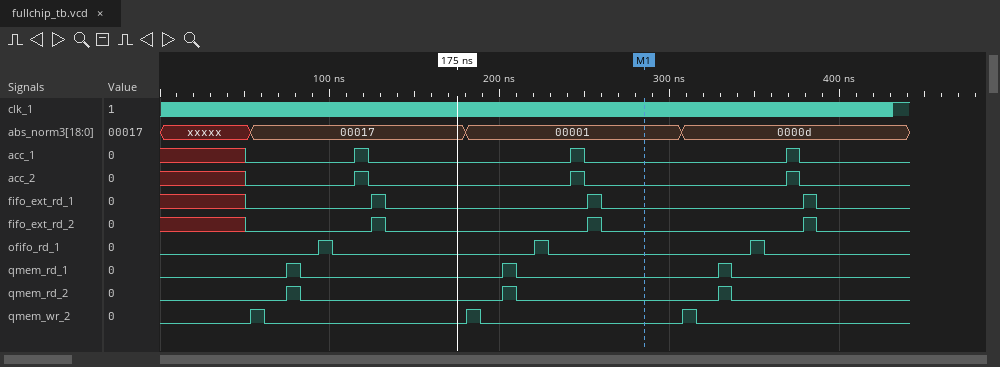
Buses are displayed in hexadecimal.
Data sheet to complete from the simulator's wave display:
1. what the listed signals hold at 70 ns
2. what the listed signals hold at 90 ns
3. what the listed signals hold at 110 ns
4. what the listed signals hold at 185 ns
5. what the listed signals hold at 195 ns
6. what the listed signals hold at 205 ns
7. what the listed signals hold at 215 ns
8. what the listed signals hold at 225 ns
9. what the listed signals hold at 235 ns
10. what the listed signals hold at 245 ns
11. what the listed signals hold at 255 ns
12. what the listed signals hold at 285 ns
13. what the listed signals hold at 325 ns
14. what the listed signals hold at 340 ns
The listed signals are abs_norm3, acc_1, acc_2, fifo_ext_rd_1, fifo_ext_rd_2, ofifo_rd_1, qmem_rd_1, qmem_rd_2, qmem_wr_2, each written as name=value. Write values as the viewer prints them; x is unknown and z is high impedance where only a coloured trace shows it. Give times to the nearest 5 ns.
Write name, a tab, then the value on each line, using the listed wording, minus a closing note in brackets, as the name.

what the listed signals hold at 70 ns	abs_norm3=00017, acc_1=0, acc_2=0, fifo_ext_rd_1=0, fifo_ext_rd_2=0, ofifo_rd_1=0, qmem_rd_1=0, qmem_rd_2=0, qmem_wr_2=0
what the listed signals hold at 90 ns	abs_norm3=00017, acc_1=0, acc_2=0, fifo_ext_rd_1=0, fifo_ext_rd_2=0, ofifo_rd_1=0, qmem_rd_1=0, qmem_rd_2=0, qmem_wr_2=0
what the listed signals hold at 110 ns	abs_norm3=00017, acc_1=0, acc_2=0, fifo_ext_rd_1=0, fifo_ext_rd_2=0, ofifo_rd_1=0, qmem_rd_1=0, qmem_rd_2=0, qmem_wr_2=0
what the listed signals hold at 185 ns	abs_norm3=00001, acc_1=0, acc_2=0, fifo_ext_rd_1=0, fifo_ext_rd_2=0, ofifo_rd_1=0, qmem_rd_1=0, qmem_rd_2=0, qmem_wr_2=1
what the listed signals hold at 195 ns	abs_norm3=00001, acc_1=0, acc_2=0, fifo_ext_rd_1=0, fifo_ext_rd_2=0, ofifo_rd_1=0, qmem_rd_1=0, qmem_rd_2=0, qmem_wr_2=0
what the listed signals hold at 205 ns	abs_norm3=00001, acc_1=0, acc_2=0, fifo_ext_rd_1=0, fifo_ext_rd_2=0, ofifo_rd_1=0, qmem_rd_1=1, qmem_rd_2=1, qmem_wr_2=0
what the listed signals hold at 215 ns	abs_norm3=00001, acc_1=0, acc_2=0, fifo_ext_rd_1=0, fifo_ext_rd_2=0, ofifo_rd_1=0, qmem_rd_1=0, qmem_rd_2=0, qmem_wr_2=0
what the listed signals hold at 225 ns	abs_norm3=00001, acc_1=0, acc_2=0, fifo_ext_rd_1=0, fifo_ext_rd_2=0, ofifo_rd_1=1, qmem_rd_1=0, qmem_rd_2=0, qmem_wr_2=0
what the listed signals hold at 235 ns	abs_norm3=00001, acc_1=0, acc_2=0, fifo_ext_rd_1=0, fifo_ext_rd_2=0, ofifo_rd_1=0, qmem_rd_1=0, qmem_rd_2=0, qmem_wr_2=0
what the listed signals hold at 245 ns	abs_norm3=00001, acc_1=1, acc_2=1, fifo_ext_rd_1=0, fifo_ext_rd_2=0, ofifo_rd_1=0, qmem_rd_1=0, qmem_rd_2=0, qmem_wr_2=0
what the listed signals hold at 255 ns	abs_norm3=00001, acc_1=0, acc_2=0, fifo_ext_rd_1=1, fifo_ext_rd_2=1, ofifo_rd_1=0, qmem_rd_1=0, qmem_rd_2=0, qmem_wr_2=0
what the listed signals hold at 285 ns	abs_norm3=00001, acc_1=0, acc_2=0, fifo_ext_rd_1=0, fifo_ext_rd_2=0, ofifo_rd_1=0, qmem_rd_1=0, qmem_rd_2=0, qmem_wr_2=0
what the listed signals hold at 325 ns	abs_norm3=0000d, acc_1=0, acc_2=0, fifo_ext_rd_1=0, fifo_ext_rd_2=0, ofifo_rd_1=0, qmem_rd_1=0, qmem_rd_2=0, qmem_wr_2=0
what the listed signals hold at 340 ns	abs_norm3=0000d, acc_1=0, acc_2=0, fifo_ext_rd_1=0, fifo_ext_rd_2=0, ofifo_rd_1=0, qmem_rd_1=0, qmem_rd_2=0, qmem_wr_2=0
